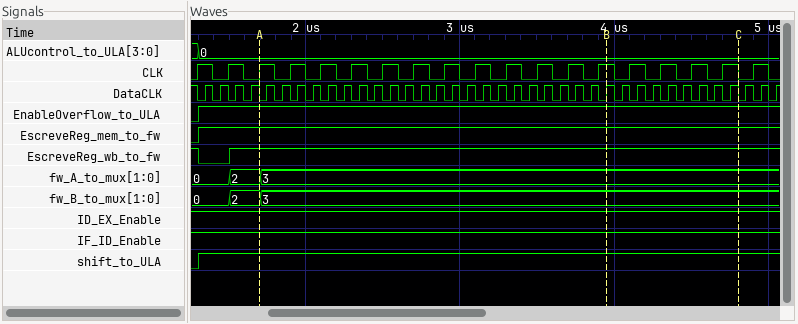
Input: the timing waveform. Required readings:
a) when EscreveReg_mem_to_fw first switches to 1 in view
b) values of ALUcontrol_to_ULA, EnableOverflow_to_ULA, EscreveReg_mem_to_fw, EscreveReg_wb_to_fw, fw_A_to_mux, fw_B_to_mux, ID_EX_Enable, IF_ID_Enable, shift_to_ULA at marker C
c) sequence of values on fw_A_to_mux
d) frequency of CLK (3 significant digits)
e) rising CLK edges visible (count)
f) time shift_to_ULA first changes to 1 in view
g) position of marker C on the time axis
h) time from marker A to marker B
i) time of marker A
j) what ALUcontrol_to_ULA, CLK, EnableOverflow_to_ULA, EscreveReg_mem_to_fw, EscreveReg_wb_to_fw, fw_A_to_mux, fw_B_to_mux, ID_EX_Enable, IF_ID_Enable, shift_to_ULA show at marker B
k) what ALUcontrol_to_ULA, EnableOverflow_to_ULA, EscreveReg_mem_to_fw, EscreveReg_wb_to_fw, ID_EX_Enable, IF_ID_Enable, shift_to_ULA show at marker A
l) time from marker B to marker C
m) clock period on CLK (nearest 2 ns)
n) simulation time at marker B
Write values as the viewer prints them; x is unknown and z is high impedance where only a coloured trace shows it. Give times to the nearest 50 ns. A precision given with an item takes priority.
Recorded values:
1300 ns
ALUcontrol_to_ULA=0, EnableOverflow_to_ULA=1, EscreveReg_mem_to_fw=1, EscreveReg_wb_to_fw=1, fw_A_to_mux=3, fw_B_to_mux=3, ID_EX_Enable=1, IF_ID_Enable=1, shift_to_ULA=1
0, 2, 3
5.00 MHz
19
1300 ns
4800 ns
2250 ns
1700 ns
ALUcontrol_to_ULA=0, CLK=1, EnableOverflow_to_ULA=1, EscreveReg_mem_to_fw=1, EscreveReg_wb_to_fw=1, fw_A_to_mux=3, fw_B_to_mux=3, ID_EX_Enable=1, IF_ID_Enable=1, shift_to_ULA=1
ALUcontrol_to_ULA=0, EnableOverflow_to_ULA=1, EscreveReg_mem_to_fw=1, EscreveReg_wb_to_fw=1, ID_EX_Enable=1, IF_ID_Enable=1, shift_to_ULA=1
850 ns
200 ns
3950 ns
